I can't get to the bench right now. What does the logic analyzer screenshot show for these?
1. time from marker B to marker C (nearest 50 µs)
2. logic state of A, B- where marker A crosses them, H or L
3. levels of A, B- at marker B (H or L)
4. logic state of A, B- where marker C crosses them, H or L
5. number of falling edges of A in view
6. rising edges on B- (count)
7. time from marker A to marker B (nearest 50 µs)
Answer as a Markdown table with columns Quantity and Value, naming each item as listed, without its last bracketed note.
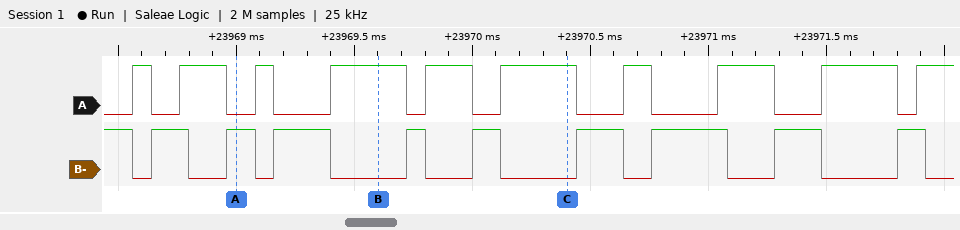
| Quantity | Value |
|---|---|
| time from marker B to marker C | 800 µs |
| logic state of A, B- where marker A crosses them, H or L | A=L, B-=H |
| levels of A, B- at marker B | A=H, B-=L |
| logic state of A, B- where marker C crosses them, H or L | A=H, B-=L |
| number of falling edges of A in view | 9 |
| rising edges on B- | 9 |
| time from marker A to marker B | 600 µs |
